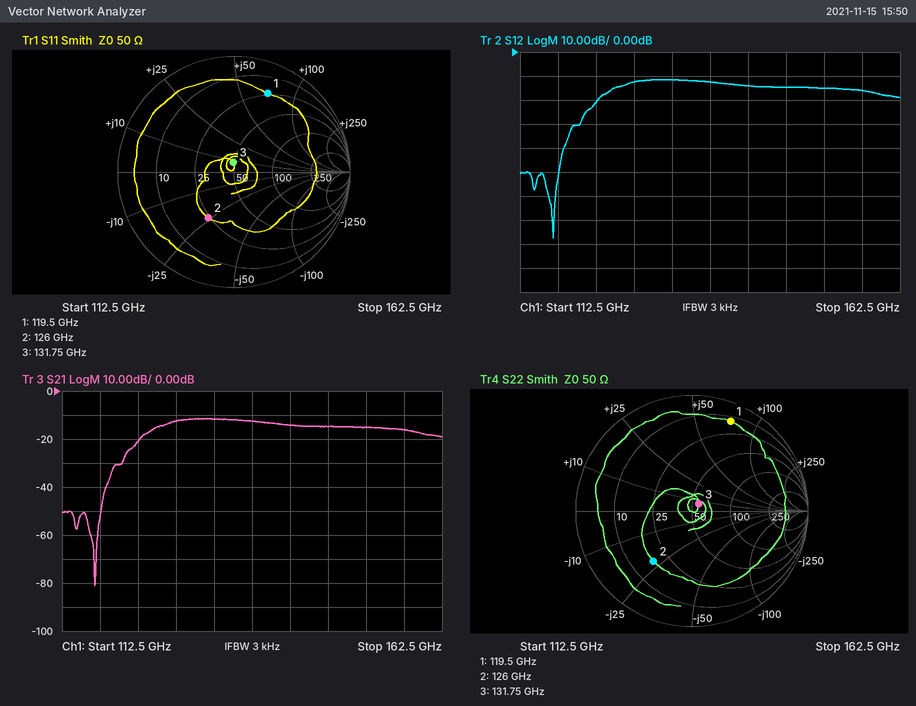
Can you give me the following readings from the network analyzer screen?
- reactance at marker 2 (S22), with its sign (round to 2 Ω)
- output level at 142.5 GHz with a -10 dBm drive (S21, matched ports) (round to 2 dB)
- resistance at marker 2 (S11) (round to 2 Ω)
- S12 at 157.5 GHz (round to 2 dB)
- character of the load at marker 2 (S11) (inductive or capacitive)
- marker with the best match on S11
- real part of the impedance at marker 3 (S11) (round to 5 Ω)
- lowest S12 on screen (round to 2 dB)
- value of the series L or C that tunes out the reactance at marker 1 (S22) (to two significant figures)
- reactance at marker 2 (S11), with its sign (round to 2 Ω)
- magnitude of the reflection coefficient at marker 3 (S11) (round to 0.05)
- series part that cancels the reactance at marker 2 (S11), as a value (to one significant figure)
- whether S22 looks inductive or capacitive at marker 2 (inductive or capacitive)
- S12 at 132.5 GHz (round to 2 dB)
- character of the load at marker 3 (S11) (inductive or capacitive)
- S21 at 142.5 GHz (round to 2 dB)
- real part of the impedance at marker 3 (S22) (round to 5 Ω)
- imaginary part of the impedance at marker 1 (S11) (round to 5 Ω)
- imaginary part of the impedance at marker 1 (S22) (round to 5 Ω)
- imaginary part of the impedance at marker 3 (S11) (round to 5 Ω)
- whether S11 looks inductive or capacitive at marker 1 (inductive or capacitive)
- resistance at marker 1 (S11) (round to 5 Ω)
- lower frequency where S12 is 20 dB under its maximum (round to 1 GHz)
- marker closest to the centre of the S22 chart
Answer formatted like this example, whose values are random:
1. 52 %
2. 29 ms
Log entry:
1. -22 Ω
2. -24 dBm
3. 24 Ω
4. -16 dB
5. capacitive
6. marker 3
7. 50 Ω
8. -78 dB
9. 18 fF
10. -24 Ω
11. 0.10
12. 30 pH
13. capacitive
14. -12 dB
15. inductive
16. -14 dB
17. 55 Ω
18. +70 Ω
19. +75 Ω
20. +10 Ω
21. inductive
22. 25 Ω
23. 119 GHz
24. marker 3
